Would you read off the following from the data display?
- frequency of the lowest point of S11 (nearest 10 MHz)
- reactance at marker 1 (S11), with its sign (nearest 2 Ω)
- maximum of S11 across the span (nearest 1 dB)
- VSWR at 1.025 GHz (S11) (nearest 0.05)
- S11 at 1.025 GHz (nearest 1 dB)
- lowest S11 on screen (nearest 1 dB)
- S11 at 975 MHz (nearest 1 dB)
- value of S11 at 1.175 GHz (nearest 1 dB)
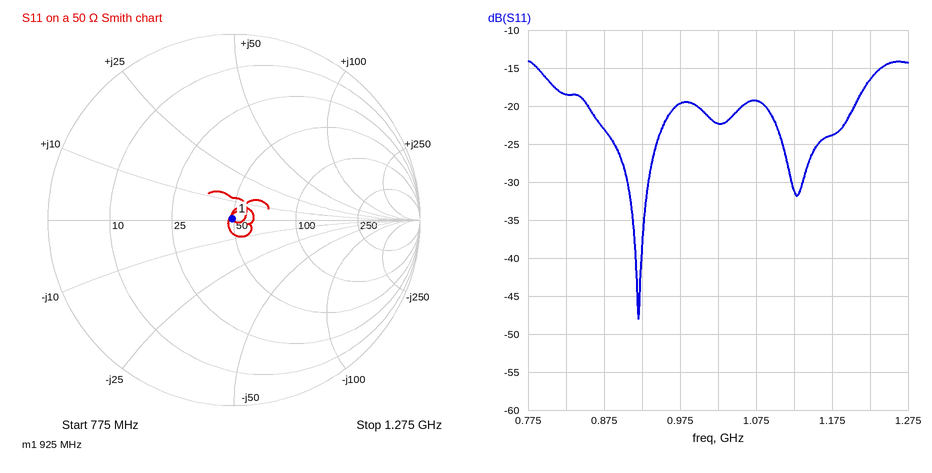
920 MHz
0 Ω
-14 dB
1.15
-22 dB
-48 dB
-20 dB
-24 dB
